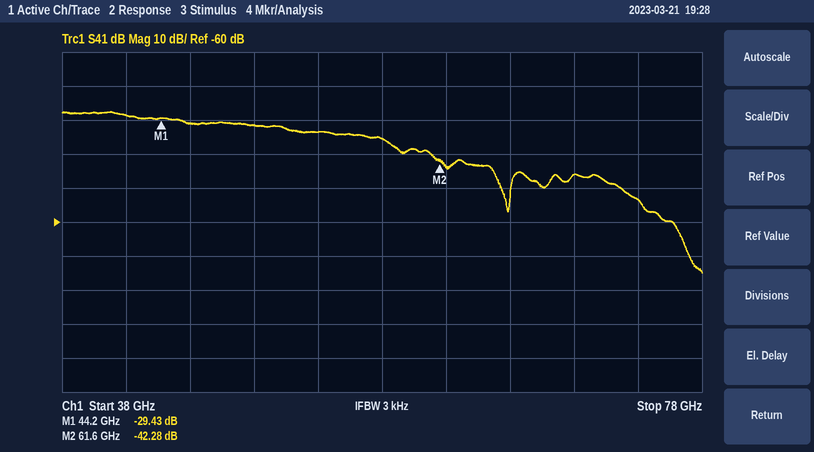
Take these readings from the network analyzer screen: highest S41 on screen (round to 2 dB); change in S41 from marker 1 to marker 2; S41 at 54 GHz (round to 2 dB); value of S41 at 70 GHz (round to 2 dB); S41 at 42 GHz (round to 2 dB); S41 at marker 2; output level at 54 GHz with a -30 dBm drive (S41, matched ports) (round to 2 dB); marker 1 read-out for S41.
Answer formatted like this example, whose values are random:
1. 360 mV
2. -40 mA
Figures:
1. -28 dB
2. -12.85 dB
3. -34 dB
4. -46 dB
5. -28 dB
6. -42.28 dB
7. -64 dBm
8. -29.43 dB
